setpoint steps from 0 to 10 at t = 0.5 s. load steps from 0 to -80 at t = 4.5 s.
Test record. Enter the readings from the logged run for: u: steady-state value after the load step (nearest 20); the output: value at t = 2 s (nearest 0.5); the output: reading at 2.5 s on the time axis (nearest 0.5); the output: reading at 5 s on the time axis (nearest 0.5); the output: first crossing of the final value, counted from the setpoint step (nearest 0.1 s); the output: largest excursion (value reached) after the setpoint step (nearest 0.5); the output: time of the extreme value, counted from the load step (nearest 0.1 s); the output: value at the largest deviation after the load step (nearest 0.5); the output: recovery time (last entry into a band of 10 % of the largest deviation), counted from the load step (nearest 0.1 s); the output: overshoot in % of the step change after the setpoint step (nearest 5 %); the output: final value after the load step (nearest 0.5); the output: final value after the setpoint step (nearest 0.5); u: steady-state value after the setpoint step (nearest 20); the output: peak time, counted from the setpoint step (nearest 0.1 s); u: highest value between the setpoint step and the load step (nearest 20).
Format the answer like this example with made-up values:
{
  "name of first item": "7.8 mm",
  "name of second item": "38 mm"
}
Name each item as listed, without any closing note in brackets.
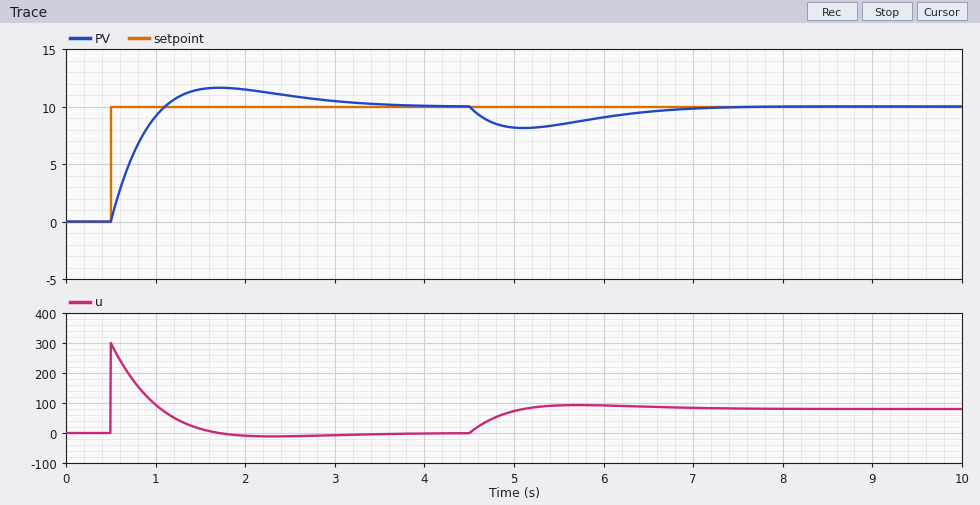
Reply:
{
  "u: steady-state value after the load step": "80",
  "the output: value at t = 2 s": "11.5",
  "the output: reading at 2.5 s on the time axis": "11.0",
  "the output: reading at 5 s on the time axis": "8.0",
  "the output: first crossing of the final value, counted from the setpoint step": "0.6 s",
  "the output: largest excursion (value reached) after the setpoint step": "11.5",
  "the output: time of the extreme value, counted from the load step": "0.6 s",
  "the output: value at the largest deviation after the load step": "8.0",
  "the output: recovery time (last entry into a band of 10 % of the largest deviation), counted from the load step": "2.5 s",
  "the output: overshoot in % of the step change after the setpoint step": "15 %",
  "the output: final value after the load step": "10.0",
  "the output: final value after the setpoint step": "10.0",
  "u: steady-state value after the setpoint step": "0",
  "the output: peak time, counted from the setpoint step": "1.2 s",
  "u: highest value between the setpoint step and the load step": "300"
}
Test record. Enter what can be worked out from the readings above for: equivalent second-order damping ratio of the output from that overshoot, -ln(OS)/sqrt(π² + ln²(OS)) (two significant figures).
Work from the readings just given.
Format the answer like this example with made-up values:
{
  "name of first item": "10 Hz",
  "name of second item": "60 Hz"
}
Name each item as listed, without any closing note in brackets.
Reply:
{
  "equivalent second-order damping ratio of the output from that overshoot, -ln(OS)/sqrt(π² + ln²(OS))": "0.52"
}
